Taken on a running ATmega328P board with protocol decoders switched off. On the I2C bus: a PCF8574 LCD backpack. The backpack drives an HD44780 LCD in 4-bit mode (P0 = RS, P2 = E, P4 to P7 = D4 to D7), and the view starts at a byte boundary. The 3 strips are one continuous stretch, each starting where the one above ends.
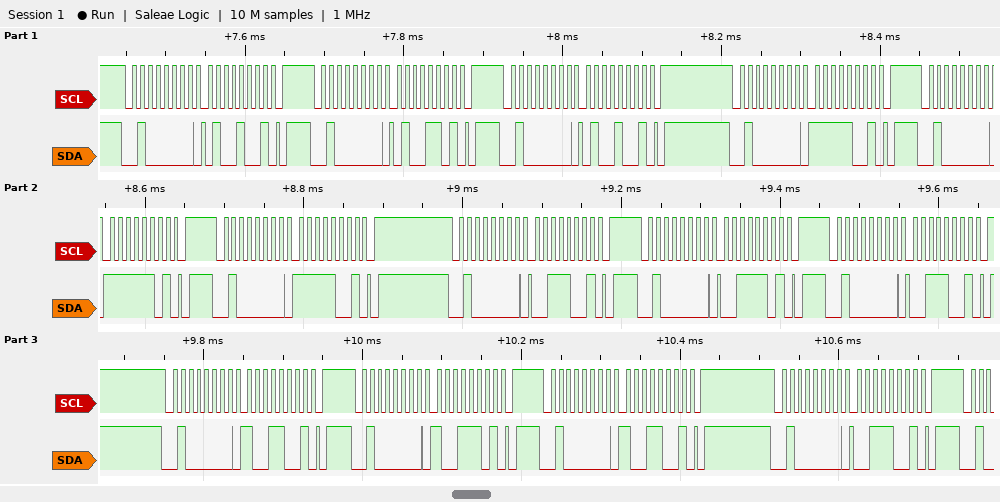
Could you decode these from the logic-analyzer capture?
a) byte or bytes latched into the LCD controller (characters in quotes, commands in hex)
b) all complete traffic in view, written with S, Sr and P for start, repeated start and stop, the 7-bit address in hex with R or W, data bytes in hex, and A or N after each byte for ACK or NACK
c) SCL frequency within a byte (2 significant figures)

'O' '9'
S 20W A 49 A P S 20W A 4D A P S 20W A 49 A P S 20W A F9 A P S 20W A FD A P S 20W A F9 A P S 20W A 39 A P S 20W A 3D A P S 20W A 39 A P S 20W A 99 A P S 20W A 9D A P S 20W A 99 A P S 20W A 39 A P
100 kHz
